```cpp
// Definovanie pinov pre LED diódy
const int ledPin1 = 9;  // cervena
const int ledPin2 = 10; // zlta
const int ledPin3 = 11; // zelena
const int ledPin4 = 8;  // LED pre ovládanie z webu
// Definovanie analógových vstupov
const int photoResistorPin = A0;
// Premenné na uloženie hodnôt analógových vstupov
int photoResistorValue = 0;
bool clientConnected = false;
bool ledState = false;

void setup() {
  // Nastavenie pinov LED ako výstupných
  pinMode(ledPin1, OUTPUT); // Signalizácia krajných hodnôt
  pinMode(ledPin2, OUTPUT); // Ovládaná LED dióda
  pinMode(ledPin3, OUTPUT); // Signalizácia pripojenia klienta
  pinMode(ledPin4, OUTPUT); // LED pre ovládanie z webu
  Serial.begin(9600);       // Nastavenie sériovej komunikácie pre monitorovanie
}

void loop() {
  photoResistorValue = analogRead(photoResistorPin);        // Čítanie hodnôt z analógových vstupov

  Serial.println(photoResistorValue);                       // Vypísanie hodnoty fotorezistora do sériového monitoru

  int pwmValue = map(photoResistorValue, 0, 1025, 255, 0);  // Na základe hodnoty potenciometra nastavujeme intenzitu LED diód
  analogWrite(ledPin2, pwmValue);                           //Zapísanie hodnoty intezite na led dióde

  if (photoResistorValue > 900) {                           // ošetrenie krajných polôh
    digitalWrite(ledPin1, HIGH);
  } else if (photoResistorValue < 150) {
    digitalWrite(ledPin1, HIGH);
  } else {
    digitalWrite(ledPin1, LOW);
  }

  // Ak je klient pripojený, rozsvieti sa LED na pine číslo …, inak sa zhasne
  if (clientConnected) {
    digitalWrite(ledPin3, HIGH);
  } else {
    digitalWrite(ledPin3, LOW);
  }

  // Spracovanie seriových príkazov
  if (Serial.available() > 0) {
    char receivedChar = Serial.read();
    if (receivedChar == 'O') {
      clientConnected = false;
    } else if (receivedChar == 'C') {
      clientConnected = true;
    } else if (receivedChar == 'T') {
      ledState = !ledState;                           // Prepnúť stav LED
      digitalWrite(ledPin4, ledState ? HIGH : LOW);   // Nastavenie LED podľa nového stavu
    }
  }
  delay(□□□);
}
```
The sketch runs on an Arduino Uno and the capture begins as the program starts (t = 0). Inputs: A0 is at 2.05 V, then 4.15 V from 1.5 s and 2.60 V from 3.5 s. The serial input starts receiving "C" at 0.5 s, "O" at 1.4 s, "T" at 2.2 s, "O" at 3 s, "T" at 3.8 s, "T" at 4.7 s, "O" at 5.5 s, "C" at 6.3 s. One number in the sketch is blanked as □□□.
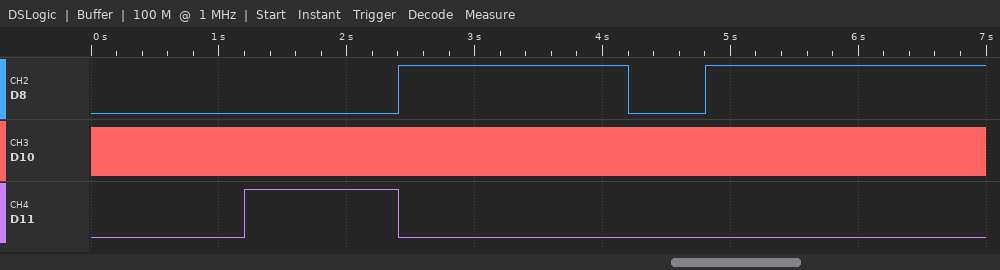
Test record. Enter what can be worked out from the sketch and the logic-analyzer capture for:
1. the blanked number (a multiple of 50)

600
